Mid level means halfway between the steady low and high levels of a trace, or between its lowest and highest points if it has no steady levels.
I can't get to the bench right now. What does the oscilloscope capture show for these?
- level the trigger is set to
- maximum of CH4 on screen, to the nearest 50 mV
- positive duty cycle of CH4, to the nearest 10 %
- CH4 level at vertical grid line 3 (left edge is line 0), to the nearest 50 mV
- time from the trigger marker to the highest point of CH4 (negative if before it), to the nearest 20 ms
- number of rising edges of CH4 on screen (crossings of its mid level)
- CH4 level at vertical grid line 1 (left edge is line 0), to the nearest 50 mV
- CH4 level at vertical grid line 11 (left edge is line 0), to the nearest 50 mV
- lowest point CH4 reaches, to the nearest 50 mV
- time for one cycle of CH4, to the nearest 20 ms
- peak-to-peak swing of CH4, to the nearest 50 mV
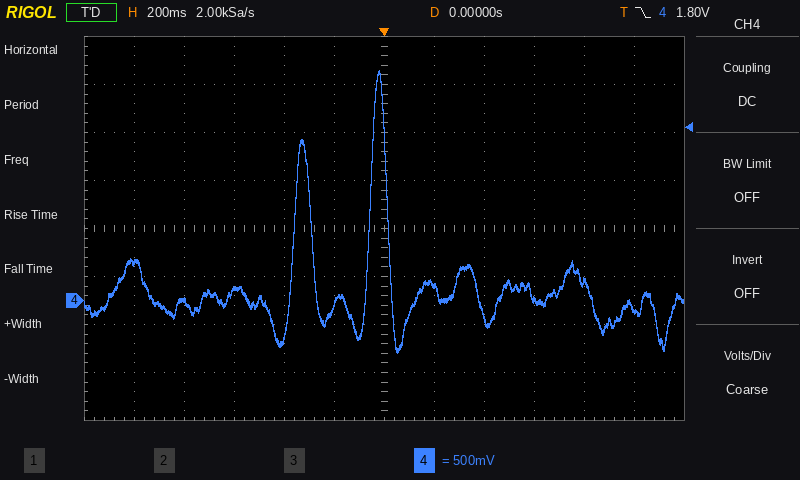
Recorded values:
1.80 V
2.40 V
20 %
100 mV
-20 ms
2
400 mV
-100 mV
-550 mV
300 ms
2.95 V
